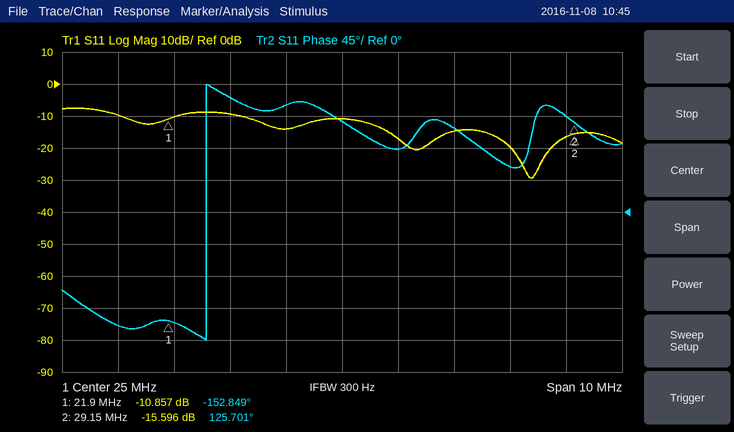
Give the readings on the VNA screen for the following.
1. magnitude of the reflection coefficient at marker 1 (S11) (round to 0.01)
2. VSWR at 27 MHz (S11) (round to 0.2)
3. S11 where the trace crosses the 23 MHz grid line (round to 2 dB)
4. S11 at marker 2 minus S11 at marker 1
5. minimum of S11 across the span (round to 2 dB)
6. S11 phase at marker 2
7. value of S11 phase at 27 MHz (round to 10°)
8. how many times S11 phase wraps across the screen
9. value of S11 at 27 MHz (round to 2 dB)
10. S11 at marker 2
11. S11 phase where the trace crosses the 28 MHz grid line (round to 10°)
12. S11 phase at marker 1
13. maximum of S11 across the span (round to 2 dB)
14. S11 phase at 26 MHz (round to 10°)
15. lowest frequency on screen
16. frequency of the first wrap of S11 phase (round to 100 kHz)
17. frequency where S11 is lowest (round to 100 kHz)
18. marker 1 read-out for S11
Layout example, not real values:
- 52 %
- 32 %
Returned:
- 0.29
- 1.4
- -10 dB
- -4.739 dB
- -30 dB
- 125.701°
- 120°
- 1
- -14 dB
- -15.596 dB
- 60°
- -152.849°
- -8 dB
- 90°
- 20 MHz
- 22.6 MHz
- 28.4 MHz
- -10.857 dB
